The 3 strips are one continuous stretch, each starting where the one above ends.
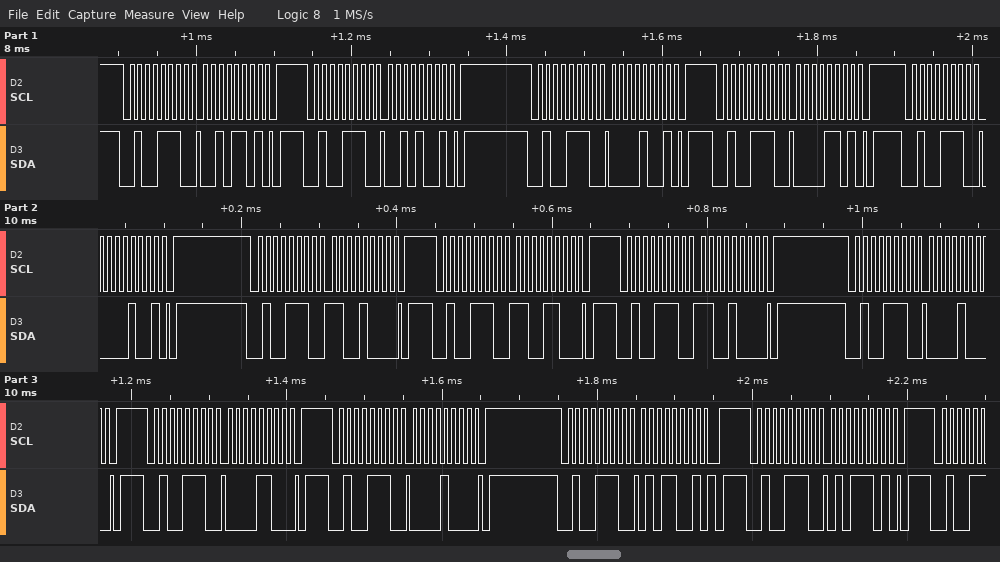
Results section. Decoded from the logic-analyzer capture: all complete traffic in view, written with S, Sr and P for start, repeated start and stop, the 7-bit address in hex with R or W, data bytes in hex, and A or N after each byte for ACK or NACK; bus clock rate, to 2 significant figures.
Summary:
S 27W A 2D A P S 27W A 29 A P S 27W A 09 A P S 27W A 0D A P S 27W A 09 A P S 27W A C8 A P S 27W A CC A P S 27W A C8 A P S 27W A 08 A P S 27W A 0C A P S 27W A 08 A P S 27W A 59 A P S 27W A 5D A P
100 kHz
